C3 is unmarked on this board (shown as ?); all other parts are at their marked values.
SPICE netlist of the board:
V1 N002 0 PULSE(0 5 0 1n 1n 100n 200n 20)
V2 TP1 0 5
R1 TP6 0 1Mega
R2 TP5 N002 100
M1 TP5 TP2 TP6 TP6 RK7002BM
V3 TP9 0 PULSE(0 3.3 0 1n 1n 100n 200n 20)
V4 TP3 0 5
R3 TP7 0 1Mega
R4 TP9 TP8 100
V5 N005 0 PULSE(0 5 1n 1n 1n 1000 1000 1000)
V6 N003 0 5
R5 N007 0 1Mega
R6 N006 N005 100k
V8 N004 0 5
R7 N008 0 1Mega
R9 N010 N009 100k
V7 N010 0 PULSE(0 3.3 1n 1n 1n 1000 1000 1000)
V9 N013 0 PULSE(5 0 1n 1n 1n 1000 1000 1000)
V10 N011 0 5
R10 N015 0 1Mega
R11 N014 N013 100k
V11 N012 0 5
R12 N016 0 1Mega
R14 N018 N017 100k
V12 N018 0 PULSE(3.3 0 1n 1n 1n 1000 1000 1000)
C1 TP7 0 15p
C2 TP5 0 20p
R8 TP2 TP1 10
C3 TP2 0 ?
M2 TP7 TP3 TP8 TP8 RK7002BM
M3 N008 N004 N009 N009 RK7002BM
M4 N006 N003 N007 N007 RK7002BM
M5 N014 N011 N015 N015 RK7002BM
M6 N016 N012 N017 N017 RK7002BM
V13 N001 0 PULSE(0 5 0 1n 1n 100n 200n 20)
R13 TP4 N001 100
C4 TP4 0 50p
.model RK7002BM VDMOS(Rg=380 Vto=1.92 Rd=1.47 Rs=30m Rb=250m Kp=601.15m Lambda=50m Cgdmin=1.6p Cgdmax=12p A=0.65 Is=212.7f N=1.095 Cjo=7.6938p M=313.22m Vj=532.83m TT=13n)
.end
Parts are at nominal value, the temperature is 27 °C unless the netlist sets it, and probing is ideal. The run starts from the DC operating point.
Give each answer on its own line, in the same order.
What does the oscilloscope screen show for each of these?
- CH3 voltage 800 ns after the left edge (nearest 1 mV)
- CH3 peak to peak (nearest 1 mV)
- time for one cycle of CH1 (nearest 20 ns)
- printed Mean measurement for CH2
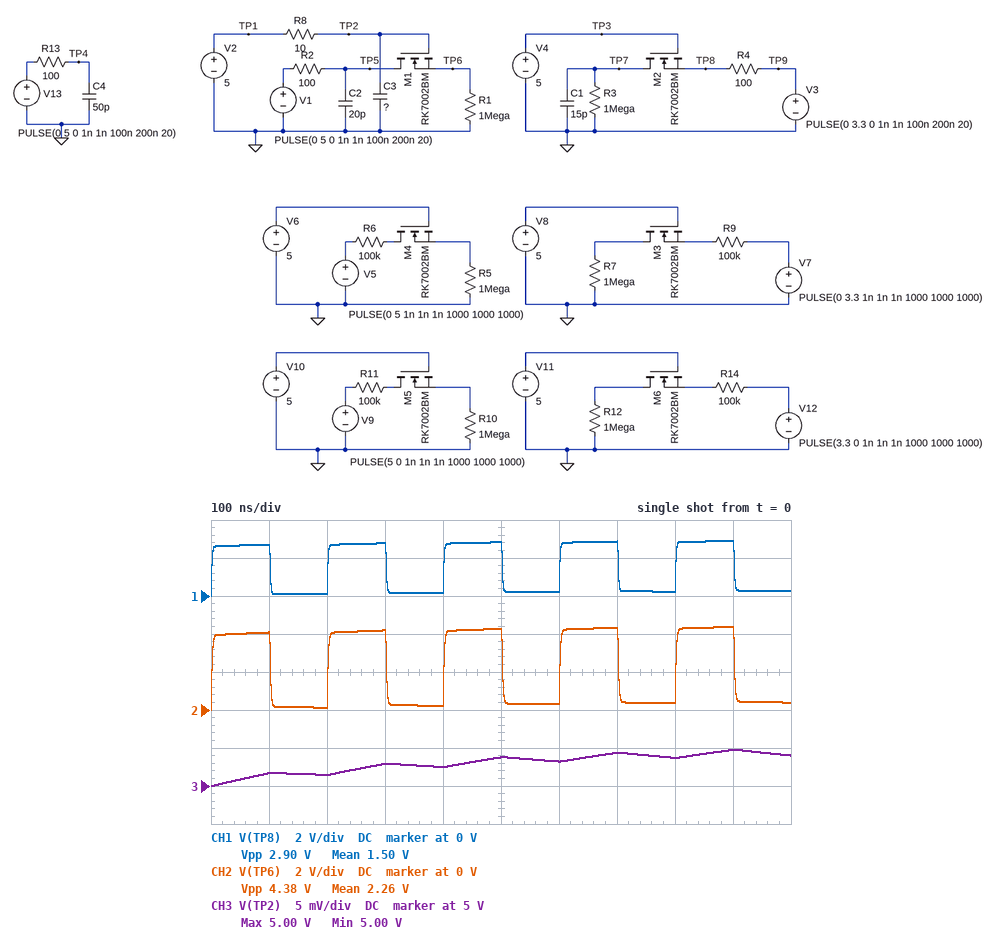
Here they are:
5.004 V
5 mV
200 ns
2.26 V
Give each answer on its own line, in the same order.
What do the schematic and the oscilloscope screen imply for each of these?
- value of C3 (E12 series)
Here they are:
560 nF
